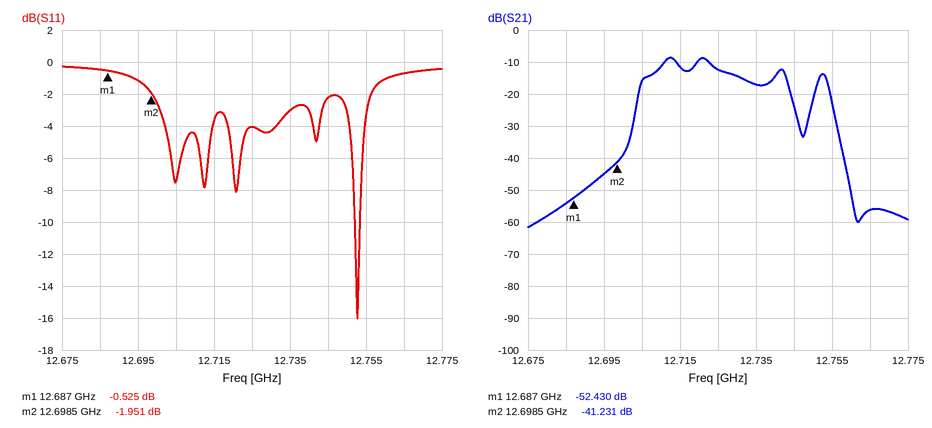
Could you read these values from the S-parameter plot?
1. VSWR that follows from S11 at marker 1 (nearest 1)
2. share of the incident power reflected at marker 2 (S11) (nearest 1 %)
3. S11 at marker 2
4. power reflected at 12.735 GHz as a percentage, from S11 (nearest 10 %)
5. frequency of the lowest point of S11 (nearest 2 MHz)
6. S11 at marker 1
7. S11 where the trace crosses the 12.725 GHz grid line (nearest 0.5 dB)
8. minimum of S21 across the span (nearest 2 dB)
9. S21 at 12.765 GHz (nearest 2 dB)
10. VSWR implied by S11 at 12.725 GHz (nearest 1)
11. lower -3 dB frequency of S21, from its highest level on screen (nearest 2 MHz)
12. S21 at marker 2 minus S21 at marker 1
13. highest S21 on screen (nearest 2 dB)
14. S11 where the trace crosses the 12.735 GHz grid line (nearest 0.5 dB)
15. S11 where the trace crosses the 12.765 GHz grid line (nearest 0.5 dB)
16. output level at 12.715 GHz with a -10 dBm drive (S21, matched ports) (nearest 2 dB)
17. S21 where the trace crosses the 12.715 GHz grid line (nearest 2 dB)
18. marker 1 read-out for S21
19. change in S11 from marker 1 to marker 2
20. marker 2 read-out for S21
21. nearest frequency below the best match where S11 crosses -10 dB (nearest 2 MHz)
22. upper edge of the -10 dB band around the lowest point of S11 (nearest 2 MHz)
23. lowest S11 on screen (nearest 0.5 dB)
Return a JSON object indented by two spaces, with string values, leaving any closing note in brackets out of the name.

{
  "VSWR that follows from S11 at marker 1": "33",
  "share of the incident power reflected at marker 2 (S11)": "64 %",
  "S11 at marker 2": "-1.951 dB",
  "power reflected at 12.735 GHz as a percentage, from S11": "50 %",
  "frequency of the lowest point of S11": "12.752 GHz",
  "S11 at marker 1": "-0.525 dB",
  "S11 where the trace crosses the 12.725 GHz grid line": "-4.0 dB",
  "minimum of S21 across the span": "-62 dB",
  "S21 at 12.765 GHz": "-56 dB",
  "VSWR implied by S11 at 12.725 GHz": "4",
  "lower -3 dB frequency of S21, from its highest level on screen": "12.710 GHz",
  "S21 at marker 2 minus S21 at marker 1": "11.199 dB",
  "highest S21 on screen": "-8 dB",
  "S11 where the trace crosses the 12.735 GHz grid line": "-3.0 dB",
  "S11 where the trace crosses the 12.765 GHz grid line": "-0.5 dB",
  "output level at 12.715 GHz with a -10 dBm drive (S21, matched ports)": "-22 dBm",
  "S21 where the trace crosses the 12.715 GHz grid line": "-12 dB",
  "marker 1 read-out for S21": "-52.430 dB",
  "change in S11 from marker 1 to marker 2": "-1.426 dB",
  "marker 2 read-out for S21": "-41.231 dB",
  "nearest frequency below the best match where S11 crosses -10 dB": "12.752 GHz",
  "upper edge of the -10 dB band around the lowest point of S11": "12.754 GHz",
  "lowest S11 on screen": "-16.0 dB"
}
